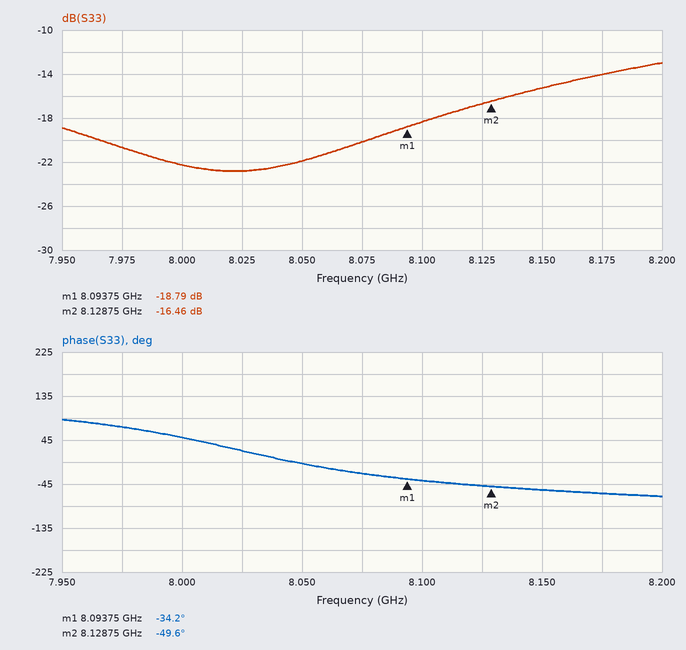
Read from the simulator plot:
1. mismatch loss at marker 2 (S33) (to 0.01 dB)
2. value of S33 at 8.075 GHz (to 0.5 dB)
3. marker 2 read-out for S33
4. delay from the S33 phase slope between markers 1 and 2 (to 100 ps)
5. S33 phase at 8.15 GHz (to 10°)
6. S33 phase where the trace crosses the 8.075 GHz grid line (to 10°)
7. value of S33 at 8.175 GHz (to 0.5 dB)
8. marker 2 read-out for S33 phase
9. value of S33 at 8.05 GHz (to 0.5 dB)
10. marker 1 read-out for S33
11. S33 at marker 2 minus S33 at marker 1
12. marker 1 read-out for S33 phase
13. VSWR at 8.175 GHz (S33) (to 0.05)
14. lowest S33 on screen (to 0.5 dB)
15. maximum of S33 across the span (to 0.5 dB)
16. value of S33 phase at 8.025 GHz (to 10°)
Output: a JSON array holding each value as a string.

["0.10 dB", "-20.0 dB", "-16.46 dB", "1.2 ns", "-60°", "-20°", "-14.0 dB", "-49.6°", "-22.0 dB", "-18.79 dB", "2.33 dB", "-34.2°", "1.50", "-23.0 dB", "-13.0 dB", "20°"]
